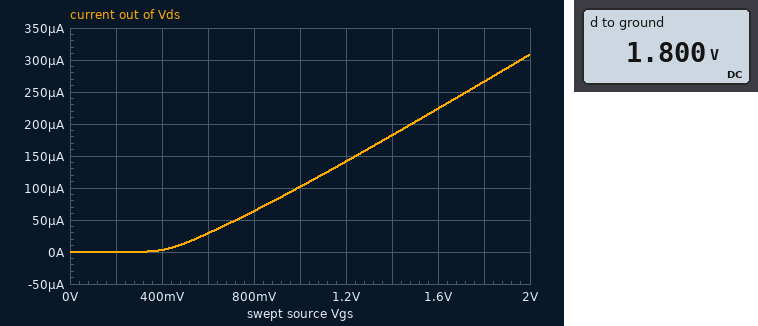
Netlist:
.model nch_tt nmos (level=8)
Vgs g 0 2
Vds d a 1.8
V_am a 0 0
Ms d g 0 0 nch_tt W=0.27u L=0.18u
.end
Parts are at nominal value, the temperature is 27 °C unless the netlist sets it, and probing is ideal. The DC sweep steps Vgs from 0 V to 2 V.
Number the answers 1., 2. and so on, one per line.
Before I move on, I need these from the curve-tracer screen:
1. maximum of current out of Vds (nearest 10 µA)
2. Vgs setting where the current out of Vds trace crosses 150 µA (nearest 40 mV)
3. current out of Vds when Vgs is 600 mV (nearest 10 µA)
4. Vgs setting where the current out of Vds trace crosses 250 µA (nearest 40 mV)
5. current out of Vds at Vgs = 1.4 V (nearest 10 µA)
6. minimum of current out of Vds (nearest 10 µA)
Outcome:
1. 310 µA
2. 1.24 V
3. 30 µA
4. 1.72 V
5. 180 µA
6. 0 A
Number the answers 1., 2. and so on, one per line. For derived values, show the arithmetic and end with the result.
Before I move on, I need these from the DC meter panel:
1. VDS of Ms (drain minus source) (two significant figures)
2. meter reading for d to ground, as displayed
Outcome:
1. 1.8 V = 1.8 V
2. 1.800 V
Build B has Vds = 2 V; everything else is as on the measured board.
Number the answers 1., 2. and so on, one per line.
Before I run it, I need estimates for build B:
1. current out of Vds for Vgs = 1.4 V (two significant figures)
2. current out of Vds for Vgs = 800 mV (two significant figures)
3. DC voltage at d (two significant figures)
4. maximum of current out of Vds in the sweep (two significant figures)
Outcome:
1. 190 µA
2. 66 µA
3. 2.0 V
4. 310 µA
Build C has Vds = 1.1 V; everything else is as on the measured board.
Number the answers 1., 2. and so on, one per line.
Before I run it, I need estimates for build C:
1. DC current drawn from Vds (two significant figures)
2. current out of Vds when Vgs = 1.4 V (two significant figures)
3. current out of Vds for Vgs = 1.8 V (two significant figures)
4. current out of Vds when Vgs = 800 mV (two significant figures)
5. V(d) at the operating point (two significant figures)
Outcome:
1. 280 µA
2. 170 µA
3. 240 µA
4. 57 µA
5. 1.1 V
